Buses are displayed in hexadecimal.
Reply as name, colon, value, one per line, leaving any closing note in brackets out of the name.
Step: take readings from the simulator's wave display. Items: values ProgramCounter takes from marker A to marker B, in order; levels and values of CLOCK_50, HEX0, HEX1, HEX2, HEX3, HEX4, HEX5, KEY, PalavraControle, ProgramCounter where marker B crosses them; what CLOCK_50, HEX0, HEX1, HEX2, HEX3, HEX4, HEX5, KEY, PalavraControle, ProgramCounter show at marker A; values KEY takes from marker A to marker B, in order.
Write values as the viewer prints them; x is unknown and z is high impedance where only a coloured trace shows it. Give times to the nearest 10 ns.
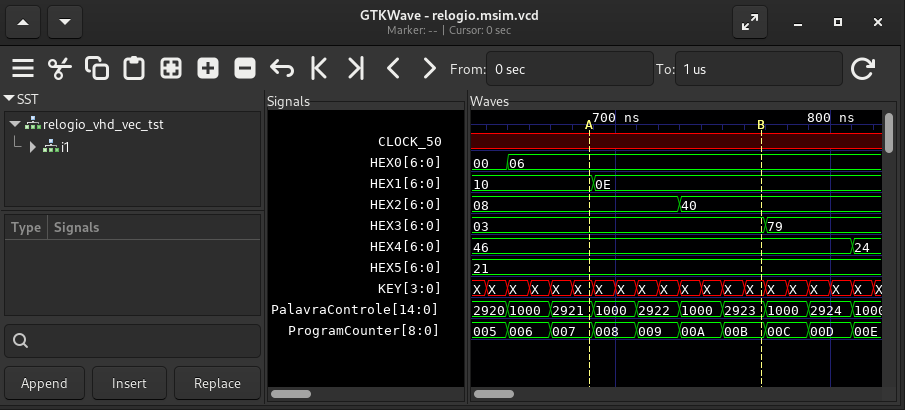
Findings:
values ProgramCounter takes from marker A to marker B, in order: 007, 008, 009, 00A, 00B
levels and values of CLOCK_50, HEX0, HEX1, HEX2, HEX3, HEX4, HEX5, KEY, PalavraControle, ProgramCounter where marker B crosses them: CLOCK_50=x, HEX0=06, HEX1=0E, HEX2=40, HEX3=03, HEX4=46, HEX5=21, KEY=X, PalavraControle=2923, ProgramCounter=00B
what CLOCK_50, HEX0, HEX1, HEX2, HEX3, HEX4, HEX5, KEY, PalavraControle, ProgramCounter show at marker A: CLOCK_50=x, HEX0=06, HEX1=10, HEX2=08, HEX3=03, HEX4=46, HEX5=21, KEY=X, PalavraControle=2921, ProgramCounter=007
values KEY takes from marker A to marker B, in order: X, X, X, X, X, X, X, X, X
